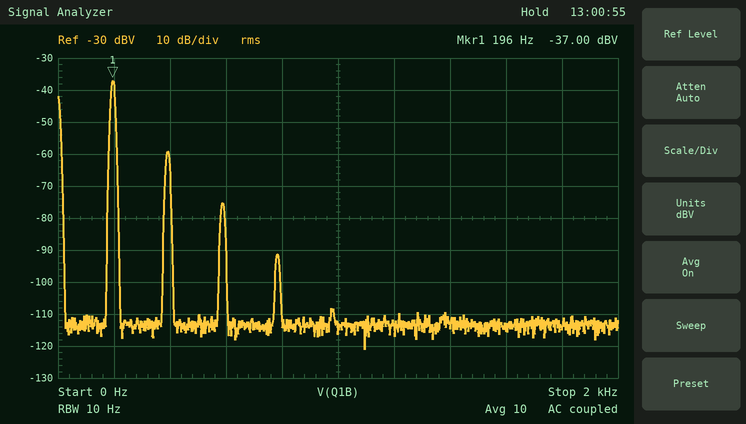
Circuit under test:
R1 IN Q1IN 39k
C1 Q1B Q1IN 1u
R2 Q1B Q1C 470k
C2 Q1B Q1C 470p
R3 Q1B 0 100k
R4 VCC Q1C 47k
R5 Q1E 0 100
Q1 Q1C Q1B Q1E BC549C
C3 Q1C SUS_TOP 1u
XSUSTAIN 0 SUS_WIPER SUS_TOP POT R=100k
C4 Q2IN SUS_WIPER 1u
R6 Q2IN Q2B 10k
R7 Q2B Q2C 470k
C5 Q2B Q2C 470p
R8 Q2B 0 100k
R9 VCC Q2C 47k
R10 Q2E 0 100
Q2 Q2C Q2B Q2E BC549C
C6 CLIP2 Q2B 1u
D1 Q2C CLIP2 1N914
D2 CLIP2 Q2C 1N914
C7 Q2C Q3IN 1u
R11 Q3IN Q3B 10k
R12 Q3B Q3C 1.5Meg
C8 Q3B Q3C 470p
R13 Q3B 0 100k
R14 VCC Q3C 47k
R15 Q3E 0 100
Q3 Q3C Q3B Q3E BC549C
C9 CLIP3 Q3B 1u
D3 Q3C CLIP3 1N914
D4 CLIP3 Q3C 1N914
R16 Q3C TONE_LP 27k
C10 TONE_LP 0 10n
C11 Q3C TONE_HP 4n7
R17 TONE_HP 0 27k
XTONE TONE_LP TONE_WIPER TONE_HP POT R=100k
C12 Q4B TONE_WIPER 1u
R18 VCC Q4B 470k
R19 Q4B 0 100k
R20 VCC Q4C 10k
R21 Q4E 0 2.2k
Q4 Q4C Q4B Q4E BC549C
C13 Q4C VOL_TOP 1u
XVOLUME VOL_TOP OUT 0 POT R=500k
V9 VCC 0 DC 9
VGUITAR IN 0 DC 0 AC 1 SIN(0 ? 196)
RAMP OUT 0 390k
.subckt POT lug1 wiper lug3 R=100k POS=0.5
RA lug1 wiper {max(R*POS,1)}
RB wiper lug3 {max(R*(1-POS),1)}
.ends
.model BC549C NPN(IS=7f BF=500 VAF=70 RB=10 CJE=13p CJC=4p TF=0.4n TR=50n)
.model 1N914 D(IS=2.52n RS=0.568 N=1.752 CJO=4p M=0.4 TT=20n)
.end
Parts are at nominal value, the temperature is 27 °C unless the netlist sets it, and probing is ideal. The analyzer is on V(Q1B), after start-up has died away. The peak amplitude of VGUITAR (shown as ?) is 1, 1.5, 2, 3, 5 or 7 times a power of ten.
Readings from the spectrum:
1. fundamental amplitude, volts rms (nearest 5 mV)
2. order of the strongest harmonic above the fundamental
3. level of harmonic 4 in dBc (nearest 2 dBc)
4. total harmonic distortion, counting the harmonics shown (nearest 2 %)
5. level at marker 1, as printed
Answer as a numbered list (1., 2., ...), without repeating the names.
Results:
1. 15 mV
2. 2
3. -54 dBc
4. 8 %
5. -37.00 dBV
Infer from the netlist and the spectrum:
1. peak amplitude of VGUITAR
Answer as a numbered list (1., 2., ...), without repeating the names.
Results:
1. 150 mV
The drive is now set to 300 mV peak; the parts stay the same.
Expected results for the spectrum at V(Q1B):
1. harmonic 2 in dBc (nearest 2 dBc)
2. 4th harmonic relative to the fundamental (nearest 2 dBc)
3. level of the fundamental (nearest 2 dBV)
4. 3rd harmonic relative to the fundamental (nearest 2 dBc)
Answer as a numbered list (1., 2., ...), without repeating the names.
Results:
1. -14 dBc
2. -32 dBc
3. -30 dBV
4. -24 dBc
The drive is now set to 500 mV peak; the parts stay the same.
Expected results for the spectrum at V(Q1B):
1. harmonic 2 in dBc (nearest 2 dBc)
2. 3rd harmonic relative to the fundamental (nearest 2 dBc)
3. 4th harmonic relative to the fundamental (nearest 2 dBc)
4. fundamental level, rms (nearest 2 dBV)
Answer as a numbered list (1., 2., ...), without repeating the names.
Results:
1. -8 dBc
2. -18 dBc
3. -28 dBc
4. -22 dBV
